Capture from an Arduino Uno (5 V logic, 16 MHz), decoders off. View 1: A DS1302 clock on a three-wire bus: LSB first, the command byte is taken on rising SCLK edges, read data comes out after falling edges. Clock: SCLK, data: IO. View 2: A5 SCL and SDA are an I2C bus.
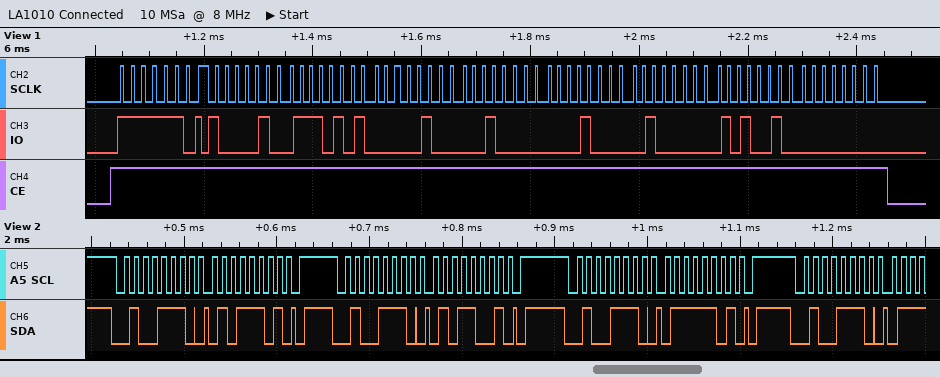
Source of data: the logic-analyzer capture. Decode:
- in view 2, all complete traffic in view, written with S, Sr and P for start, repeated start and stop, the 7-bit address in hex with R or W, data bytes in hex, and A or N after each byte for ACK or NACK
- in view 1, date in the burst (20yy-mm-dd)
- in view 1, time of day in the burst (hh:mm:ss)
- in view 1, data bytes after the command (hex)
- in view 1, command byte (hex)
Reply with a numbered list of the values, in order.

1. S 27W A 5D A P S 27W A 59 A P S 27W A 7D A P S 27W A
2. 2025-08-04
3. 10:57:21
4. 21 57 10 04 08 02 25 00
5. 0xBF
